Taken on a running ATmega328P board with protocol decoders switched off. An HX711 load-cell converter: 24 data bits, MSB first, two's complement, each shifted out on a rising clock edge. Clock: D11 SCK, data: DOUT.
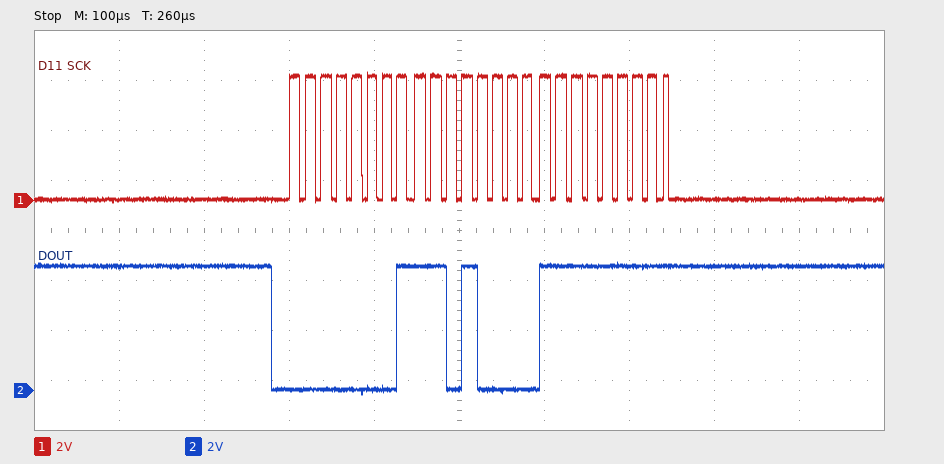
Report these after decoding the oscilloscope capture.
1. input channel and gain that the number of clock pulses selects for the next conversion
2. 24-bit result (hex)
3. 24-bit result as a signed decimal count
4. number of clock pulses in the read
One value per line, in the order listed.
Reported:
channel A, gain 128
0x01D0FF
119039
25
